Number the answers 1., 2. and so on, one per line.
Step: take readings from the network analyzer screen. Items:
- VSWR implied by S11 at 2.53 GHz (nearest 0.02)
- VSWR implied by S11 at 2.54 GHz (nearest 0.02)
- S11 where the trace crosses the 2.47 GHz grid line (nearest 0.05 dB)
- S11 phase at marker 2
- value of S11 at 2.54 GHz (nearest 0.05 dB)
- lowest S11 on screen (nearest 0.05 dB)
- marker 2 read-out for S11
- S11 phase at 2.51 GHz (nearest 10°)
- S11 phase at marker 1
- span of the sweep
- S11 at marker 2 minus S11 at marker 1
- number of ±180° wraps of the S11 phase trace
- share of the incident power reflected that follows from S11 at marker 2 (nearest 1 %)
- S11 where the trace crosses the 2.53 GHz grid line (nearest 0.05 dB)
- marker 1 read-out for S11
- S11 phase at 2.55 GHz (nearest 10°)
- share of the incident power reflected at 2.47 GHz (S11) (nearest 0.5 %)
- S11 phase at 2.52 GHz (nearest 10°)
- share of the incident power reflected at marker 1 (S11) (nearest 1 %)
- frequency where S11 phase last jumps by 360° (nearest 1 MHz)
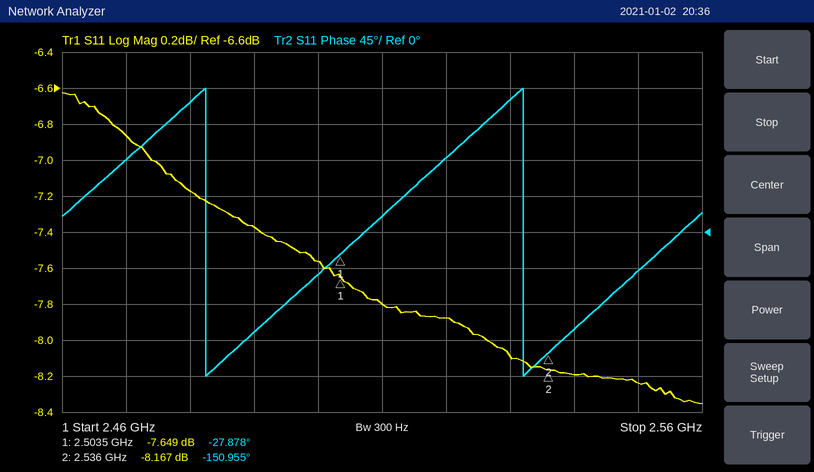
1. 2.30
2. 2.28
3. -6.85 dB
4. -150.955°
5. -8.20 dB
6. -8.35 dB
7. -8.167 dB
8. 20°
9. -27.878°
10. 100 MHz
11. -0.518 dB
12. 2
13. 15 %
14. -8.10 dB
15. -7.649 dB
16. -50°
17. 20.5 %
18. 90°
19. 17 %
20. 2.532 GHz
